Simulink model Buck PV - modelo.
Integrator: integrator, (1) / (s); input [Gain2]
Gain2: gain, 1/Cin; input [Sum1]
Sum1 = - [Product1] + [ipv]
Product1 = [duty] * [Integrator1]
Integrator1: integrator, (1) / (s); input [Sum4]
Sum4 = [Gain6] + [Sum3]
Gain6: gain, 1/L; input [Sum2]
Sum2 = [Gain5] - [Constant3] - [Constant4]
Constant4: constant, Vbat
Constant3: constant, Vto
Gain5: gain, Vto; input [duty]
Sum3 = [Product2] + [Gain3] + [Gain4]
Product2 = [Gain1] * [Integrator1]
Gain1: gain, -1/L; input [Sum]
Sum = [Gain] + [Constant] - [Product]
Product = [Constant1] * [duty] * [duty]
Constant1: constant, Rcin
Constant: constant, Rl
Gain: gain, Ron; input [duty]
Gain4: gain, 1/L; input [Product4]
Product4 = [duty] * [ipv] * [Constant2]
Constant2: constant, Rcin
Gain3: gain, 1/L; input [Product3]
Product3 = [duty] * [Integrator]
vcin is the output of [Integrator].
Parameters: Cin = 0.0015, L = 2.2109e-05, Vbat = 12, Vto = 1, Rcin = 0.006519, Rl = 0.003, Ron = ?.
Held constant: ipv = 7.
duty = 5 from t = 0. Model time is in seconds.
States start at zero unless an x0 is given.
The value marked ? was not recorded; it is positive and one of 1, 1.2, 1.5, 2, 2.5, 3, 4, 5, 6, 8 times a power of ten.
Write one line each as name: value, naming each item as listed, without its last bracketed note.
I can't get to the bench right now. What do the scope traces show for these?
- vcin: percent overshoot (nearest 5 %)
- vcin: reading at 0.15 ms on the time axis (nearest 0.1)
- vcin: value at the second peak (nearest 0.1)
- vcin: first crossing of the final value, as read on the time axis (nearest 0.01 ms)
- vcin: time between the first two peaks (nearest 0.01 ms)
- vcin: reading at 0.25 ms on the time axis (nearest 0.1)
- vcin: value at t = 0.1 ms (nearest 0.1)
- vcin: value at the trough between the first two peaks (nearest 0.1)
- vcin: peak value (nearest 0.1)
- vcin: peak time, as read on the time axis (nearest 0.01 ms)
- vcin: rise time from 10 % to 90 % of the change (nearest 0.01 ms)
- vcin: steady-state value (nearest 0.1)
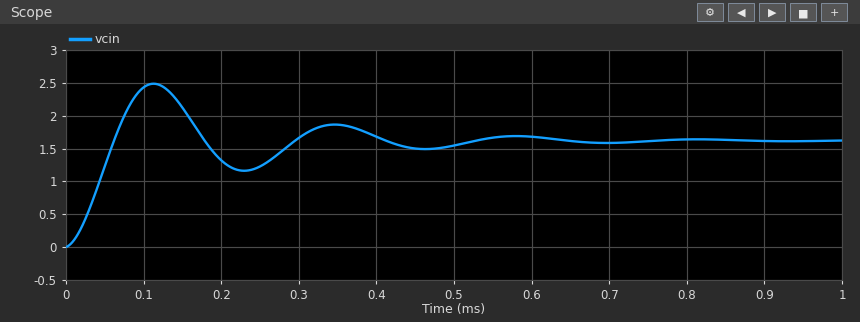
vcin: percent overshoot: 55 %
vcin: reading at 0.15 ms on the time axis: 2.1
vcin: value at the second peak: 1.9
vcin: first crossing of the final value, as read on the time axis: 0.06 ms
vcin: time between the first two peaks: 0.23 ms
vcin: reading at 0.25 ms on the time axis: 1.2
vcin: value at t = 0.1 ms: 2.4
vcin: value at the trough between the first two peaks: 1.2
vcin: peak value: 2.5
vcin: peak time, as read on the time axis: 0.11 ms
vcin: rise time from 10 % to 90 % of the change: 0.04 ms
vcin: steady-state value: 1.6
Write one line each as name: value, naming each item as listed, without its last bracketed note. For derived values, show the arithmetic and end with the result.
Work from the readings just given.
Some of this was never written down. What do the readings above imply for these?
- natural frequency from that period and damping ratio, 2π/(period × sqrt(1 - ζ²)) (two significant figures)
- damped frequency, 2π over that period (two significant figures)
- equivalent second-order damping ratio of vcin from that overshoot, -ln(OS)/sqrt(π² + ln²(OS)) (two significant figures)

natural frequency from that period and damping ratio, 2π/(period × sqrt(1 - ζ²)): 2π / (0.23 × sqrt(1 - 0.19²)) = 28 rad/ms
damped frequency, 2π over that period: 2π / 0.23 = 27 rad/ms
equivalent second-order damping ratio of vcin from that overshoot, -ln(OS)/sqrt(π² + ln²(OS)): ln(0.55) = -0.598; 0.598 / sqrt(9.870 + 0.357) = 0.19
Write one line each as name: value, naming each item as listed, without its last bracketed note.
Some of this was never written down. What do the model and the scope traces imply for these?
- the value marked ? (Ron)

the value marked ?: 0.08
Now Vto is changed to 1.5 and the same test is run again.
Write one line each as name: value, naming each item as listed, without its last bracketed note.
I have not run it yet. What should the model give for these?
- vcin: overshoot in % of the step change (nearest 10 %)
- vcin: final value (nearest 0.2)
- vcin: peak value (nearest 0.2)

vcin: overshoot in % of the step change: 50 %
vcin: final value: 1.2
vcin: peak value: 1.8
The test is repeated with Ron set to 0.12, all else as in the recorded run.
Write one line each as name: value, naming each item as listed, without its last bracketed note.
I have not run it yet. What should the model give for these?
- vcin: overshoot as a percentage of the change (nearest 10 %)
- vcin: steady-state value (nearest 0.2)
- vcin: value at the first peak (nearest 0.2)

vcin: overshoot as a percentage of the change: 30 %
vcin: steady-state value: 1.6
vcin: value at the first peak: 2.2
